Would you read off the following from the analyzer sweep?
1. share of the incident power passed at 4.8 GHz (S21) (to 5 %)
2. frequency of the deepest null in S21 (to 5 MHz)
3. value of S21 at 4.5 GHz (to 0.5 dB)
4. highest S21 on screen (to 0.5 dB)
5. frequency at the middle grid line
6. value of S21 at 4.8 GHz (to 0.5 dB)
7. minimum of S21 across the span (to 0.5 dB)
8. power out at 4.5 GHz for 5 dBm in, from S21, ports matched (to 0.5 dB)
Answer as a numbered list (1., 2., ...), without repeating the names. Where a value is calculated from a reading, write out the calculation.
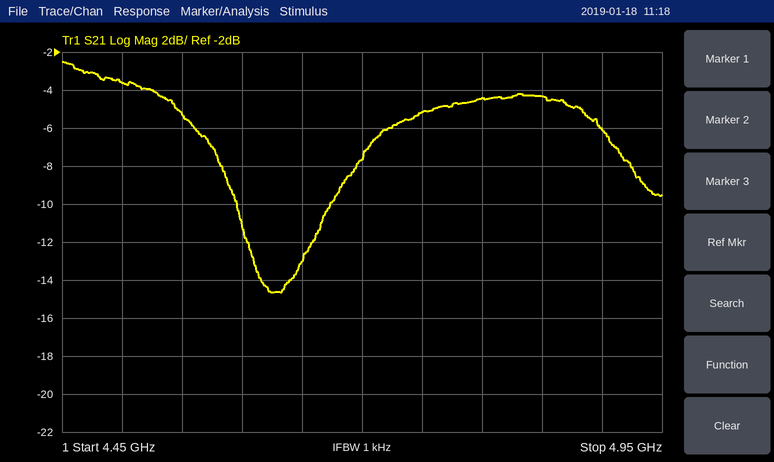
1. 10^(-4.5/10) ≈ 35 %
2. 4.625 GHz
3. -3.5 dB
4. -2.5 dB
5. 4.7 GHz
6. -4.5 dB
7. -14.5 dB
8. 5 dBm + (-3.5 dB) = 1.5 dBm
